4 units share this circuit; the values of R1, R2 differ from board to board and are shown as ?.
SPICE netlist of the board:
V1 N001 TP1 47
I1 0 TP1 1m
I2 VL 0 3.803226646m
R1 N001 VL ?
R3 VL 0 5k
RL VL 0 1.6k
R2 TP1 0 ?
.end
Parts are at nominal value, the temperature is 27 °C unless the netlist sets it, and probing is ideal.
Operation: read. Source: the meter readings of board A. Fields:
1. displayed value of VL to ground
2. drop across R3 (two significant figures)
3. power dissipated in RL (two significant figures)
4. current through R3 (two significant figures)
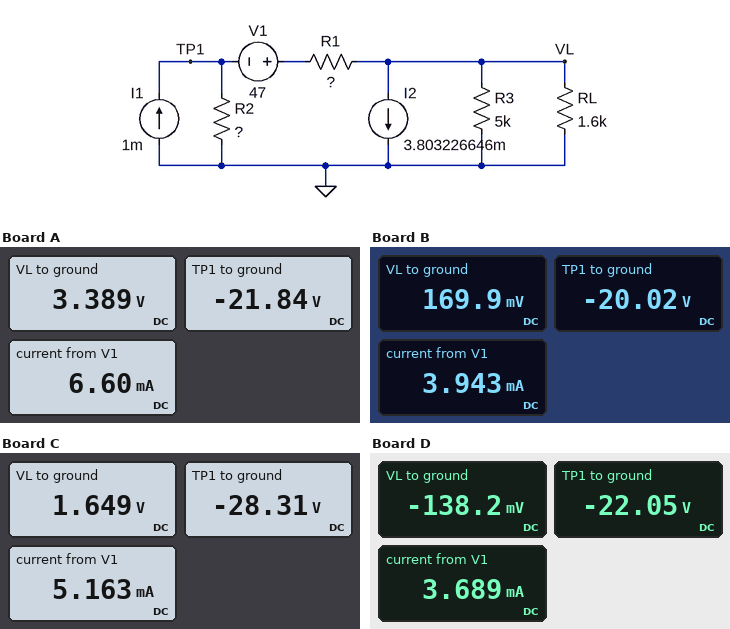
3.389 V
3.4 V
7.2 mW
680 µA
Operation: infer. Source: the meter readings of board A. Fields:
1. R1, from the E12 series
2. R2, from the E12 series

3.3 kΩ
3.9 kΩ
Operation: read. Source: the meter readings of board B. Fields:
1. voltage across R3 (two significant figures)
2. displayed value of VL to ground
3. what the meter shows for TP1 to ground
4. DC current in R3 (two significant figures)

170 mV
169.9 mV
-20.02 V
34 µA
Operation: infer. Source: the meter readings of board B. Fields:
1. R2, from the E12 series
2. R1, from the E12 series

6.8 kΩ
6.8 kΩ
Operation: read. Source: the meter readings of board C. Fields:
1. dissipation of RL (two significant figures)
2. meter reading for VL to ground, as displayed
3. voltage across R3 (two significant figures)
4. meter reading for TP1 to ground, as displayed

1.7 mW
1.649 V
1.6 V
-28.31 V
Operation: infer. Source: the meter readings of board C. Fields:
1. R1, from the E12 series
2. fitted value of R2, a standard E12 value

3.3 kΩ
6.8 kΩ
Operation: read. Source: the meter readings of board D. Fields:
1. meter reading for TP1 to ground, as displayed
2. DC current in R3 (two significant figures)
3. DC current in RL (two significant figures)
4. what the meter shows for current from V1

-22.05 V
28 µA
86 µA
3.689 mA
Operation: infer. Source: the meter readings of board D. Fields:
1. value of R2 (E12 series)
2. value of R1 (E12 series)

8.2 kΩ
6.8 kΩ
